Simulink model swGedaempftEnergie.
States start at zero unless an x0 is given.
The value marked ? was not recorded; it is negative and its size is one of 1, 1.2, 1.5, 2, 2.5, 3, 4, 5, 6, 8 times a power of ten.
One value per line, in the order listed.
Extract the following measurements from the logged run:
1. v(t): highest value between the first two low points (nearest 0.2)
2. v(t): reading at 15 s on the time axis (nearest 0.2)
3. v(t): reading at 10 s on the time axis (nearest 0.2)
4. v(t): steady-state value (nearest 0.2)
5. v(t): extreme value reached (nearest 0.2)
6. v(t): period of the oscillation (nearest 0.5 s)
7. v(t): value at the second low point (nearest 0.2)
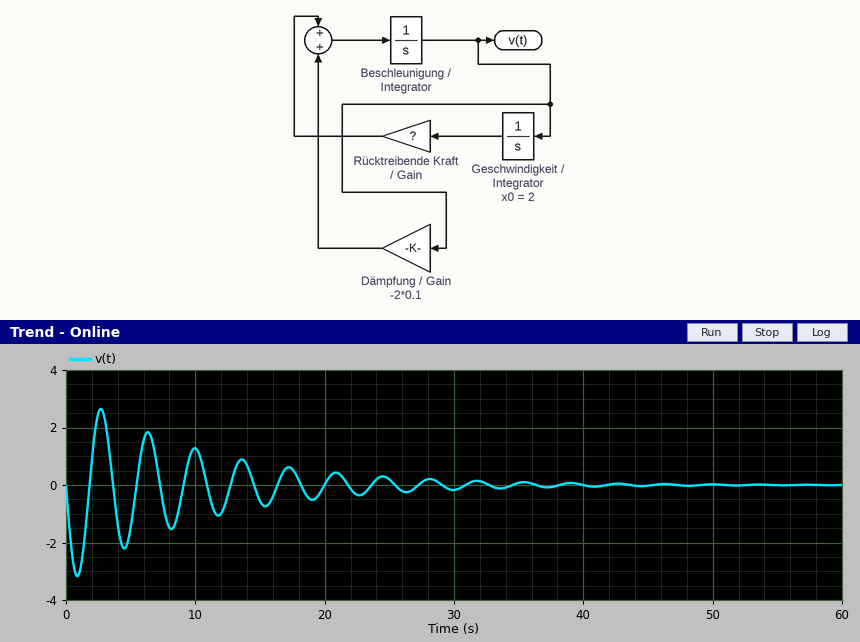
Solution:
2.6
-0.6
1.2
0.0
-3.2
3.5 s
-2.2
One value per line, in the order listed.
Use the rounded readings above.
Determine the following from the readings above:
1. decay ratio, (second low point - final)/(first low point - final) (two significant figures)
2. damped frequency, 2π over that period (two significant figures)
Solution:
0.69
1.8 rad/s
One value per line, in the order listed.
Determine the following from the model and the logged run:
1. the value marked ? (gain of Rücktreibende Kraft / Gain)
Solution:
-3
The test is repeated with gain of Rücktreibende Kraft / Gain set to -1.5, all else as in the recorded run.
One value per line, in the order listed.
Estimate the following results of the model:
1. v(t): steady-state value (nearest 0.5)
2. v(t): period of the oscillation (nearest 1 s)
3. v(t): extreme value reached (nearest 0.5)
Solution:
0.0
5 s
-2.0
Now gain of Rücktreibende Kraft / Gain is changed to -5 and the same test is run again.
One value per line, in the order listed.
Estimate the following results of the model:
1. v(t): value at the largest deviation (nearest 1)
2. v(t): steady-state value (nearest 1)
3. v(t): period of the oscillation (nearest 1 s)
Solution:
-4
0
3 s
